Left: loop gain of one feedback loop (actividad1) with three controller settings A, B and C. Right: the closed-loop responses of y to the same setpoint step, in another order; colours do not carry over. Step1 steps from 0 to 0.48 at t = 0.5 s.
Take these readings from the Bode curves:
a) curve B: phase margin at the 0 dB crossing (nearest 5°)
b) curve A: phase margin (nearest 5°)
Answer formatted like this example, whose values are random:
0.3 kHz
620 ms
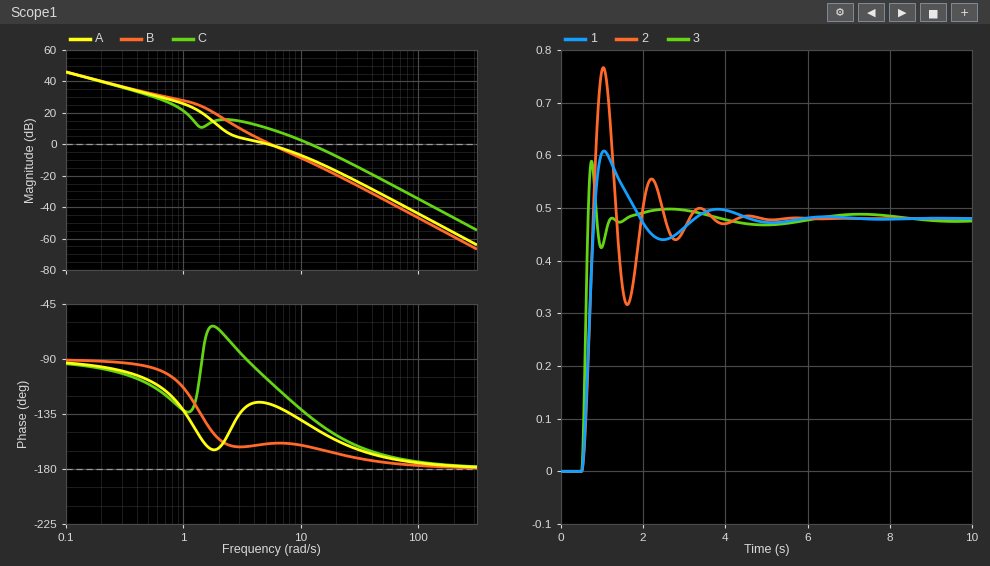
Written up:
20°
55°
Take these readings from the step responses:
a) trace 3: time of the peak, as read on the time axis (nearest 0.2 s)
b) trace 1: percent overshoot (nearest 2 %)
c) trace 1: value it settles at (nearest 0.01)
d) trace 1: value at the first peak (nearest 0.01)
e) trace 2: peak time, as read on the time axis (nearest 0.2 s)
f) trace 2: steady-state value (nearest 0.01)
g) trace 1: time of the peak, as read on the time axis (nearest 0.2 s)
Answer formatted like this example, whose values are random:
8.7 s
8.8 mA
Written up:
0.8 s
26 %
0.48
0.61
1.0 s
0.48
1.0 s
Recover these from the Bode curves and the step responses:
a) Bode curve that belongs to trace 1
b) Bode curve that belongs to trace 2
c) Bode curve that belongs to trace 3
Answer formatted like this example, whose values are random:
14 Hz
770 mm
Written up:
A
B
C
